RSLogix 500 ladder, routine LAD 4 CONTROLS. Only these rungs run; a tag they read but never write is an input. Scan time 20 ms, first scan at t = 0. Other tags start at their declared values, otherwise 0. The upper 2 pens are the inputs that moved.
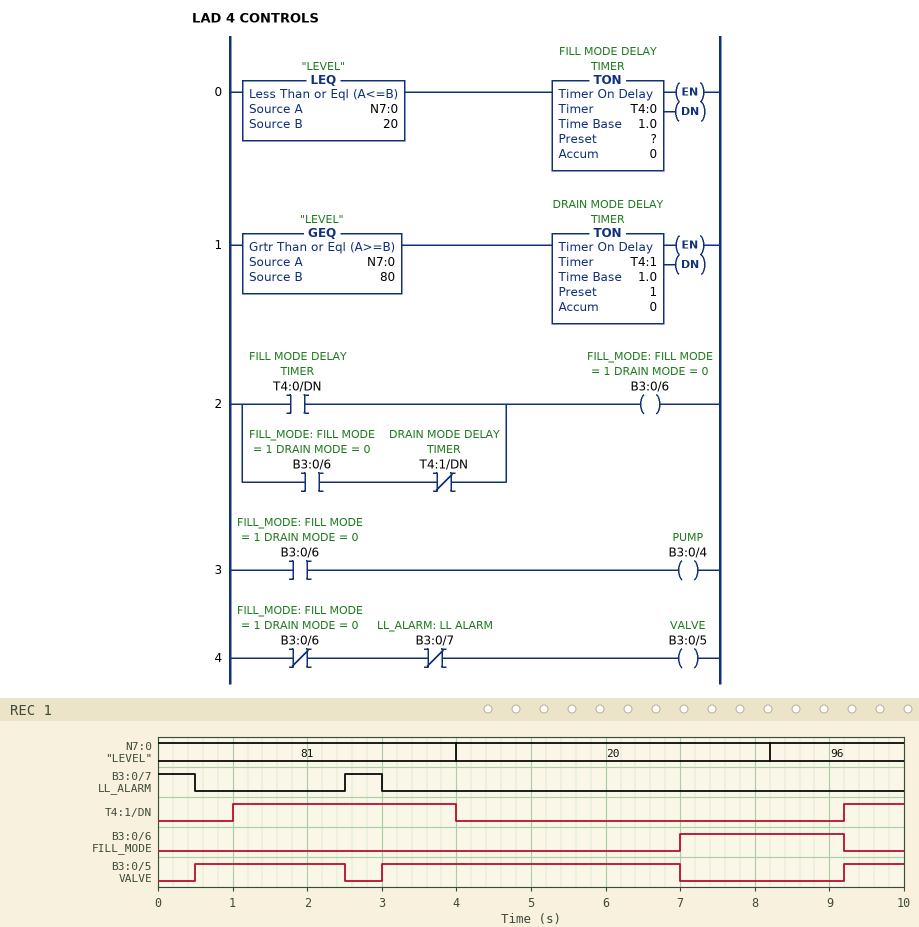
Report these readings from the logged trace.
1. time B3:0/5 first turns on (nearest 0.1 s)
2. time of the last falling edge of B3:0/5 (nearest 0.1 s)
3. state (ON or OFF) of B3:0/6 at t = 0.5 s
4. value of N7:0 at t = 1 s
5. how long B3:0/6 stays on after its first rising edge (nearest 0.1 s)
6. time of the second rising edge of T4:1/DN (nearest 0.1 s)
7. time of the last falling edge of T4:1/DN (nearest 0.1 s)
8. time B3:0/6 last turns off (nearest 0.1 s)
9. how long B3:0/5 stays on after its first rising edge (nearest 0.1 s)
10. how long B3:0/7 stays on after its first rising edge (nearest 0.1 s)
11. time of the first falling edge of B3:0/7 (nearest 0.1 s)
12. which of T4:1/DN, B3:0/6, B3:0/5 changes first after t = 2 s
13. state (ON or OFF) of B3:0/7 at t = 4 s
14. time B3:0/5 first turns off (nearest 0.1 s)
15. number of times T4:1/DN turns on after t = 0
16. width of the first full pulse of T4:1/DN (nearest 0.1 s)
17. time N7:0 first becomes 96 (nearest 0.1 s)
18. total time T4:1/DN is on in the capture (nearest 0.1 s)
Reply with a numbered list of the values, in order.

1. 0.5 s
2. 7.0 s
3. OFF
4. 81
5. 2.2 s
6. 9.2 s
7. 4.0 s
8. 9.2 s
9. 2.0 s
10. 0.5 s
11. 0.5 s
12. B3:0/5
13. OFF
14. 2.5 s
15. 2
16. 3.0 s
17. 8.2 s
18. 3.8 s
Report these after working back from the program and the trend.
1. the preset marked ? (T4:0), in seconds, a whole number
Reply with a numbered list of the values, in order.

1. 3 s
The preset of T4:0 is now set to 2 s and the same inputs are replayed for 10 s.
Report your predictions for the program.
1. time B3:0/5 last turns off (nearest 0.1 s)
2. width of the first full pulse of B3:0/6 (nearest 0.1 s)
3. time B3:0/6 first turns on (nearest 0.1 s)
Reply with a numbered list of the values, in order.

1. 6.0 s
2. 3.2 s
3. 6.0 s
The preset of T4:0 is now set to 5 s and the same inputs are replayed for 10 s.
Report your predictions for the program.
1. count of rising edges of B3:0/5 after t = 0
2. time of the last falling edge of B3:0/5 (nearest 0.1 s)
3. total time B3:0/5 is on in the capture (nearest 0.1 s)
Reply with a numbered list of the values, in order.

1. 2
2. 2.5 s
3. 9.0 s
